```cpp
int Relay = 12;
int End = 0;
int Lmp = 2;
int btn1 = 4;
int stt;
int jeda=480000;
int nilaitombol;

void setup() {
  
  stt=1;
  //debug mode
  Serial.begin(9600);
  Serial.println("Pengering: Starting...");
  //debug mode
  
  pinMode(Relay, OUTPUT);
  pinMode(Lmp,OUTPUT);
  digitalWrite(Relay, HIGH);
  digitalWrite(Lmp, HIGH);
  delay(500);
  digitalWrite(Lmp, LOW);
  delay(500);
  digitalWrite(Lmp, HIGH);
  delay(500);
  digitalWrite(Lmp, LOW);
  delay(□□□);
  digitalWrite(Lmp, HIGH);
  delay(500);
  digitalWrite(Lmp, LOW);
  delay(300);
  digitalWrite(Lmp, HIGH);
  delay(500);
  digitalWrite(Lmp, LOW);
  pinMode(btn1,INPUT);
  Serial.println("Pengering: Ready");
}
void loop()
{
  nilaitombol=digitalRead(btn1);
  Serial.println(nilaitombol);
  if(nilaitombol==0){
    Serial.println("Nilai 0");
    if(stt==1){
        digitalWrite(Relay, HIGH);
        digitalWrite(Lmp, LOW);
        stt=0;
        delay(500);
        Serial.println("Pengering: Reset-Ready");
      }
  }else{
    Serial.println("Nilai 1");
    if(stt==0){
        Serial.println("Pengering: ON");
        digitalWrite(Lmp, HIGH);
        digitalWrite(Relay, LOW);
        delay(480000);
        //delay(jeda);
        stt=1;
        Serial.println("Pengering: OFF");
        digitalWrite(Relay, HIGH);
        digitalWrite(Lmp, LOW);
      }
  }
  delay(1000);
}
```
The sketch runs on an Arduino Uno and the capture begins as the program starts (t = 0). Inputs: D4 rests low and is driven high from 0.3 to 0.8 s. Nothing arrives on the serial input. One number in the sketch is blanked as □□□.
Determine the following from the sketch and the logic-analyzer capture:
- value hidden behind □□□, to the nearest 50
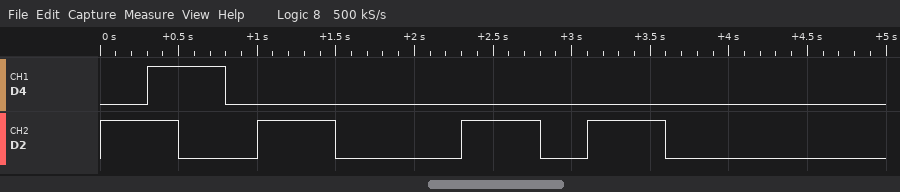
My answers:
800
